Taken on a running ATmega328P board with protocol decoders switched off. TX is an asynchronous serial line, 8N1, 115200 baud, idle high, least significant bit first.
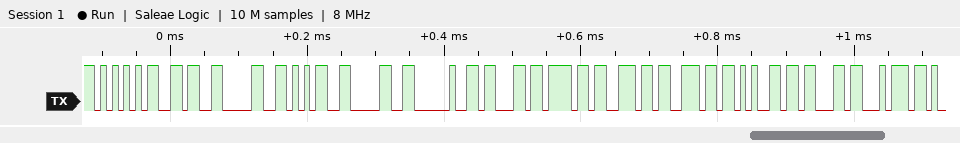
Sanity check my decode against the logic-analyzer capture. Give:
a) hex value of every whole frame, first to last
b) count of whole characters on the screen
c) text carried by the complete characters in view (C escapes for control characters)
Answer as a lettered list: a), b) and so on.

a) 55 36 30 35 30 20 63 6F 6E 6E 65 63 74
b) 13
c) "U6050 connect"
